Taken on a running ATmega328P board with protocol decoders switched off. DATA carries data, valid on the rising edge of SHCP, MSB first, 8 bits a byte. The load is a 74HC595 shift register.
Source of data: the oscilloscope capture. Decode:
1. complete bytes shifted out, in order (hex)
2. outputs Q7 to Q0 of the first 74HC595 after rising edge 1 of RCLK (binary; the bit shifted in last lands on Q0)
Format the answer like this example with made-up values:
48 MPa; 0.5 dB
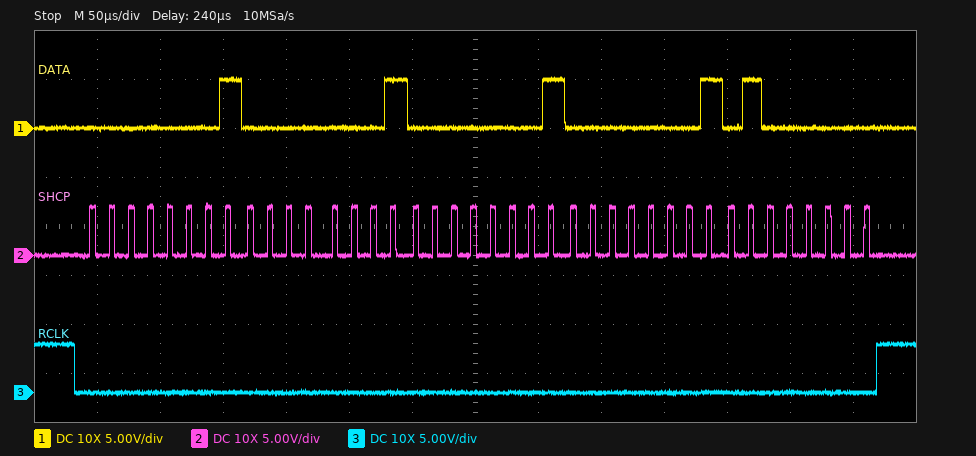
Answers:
01 01 01 01 40; 01000000
